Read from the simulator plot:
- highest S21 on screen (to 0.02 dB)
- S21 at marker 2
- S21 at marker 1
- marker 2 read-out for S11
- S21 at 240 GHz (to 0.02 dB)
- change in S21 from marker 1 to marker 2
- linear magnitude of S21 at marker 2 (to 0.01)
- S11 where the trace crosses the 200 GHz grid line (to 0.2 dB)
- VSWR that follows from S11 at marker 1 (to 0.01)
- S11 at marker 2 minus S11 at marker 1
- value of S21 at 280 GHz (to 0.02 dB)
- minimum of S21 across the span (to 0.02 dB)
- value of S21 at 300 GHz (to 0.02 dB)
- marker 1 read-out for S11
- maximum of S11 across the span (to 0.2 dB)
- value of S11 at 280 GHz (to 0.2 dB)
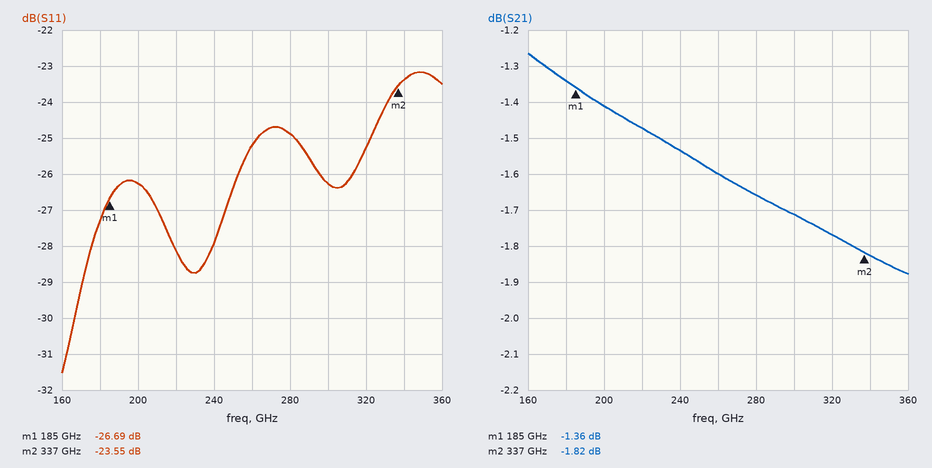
-1.26 dB
-1.82 dB
-1.36 dB
-23.55 dB
-1.54 dB
-0.46 dB
0.81
-26.2 dB
1.10
3.14 dB
-1.66 dB
-1.88 dB
-1.72 dB
-26.69 dB
-23.2 dB
-24.8 dB
